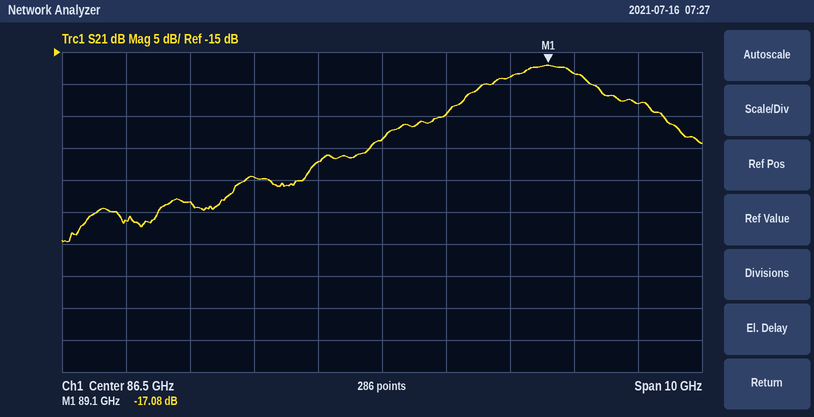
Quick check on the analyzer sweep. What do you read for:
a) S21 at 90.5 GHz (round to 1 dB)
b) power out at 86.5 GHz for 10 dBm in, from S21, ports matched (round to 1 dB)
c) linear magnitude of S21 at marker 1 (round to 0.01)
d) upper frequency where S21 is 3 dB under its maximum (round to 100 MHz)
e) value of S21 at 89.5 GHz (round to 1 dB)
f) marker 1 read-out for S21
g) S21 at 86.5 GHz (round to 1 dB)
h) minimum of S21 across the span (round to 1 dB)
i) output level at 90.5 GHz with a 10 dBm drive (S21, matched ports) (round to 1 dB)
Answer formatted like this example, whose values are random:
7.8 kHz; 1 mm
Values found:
-23 dB; -19 dBm; 0.14; 89.8 GHz; -18 dB; -17.08 dB; -29 dB; -45 dB; -13 dBm
